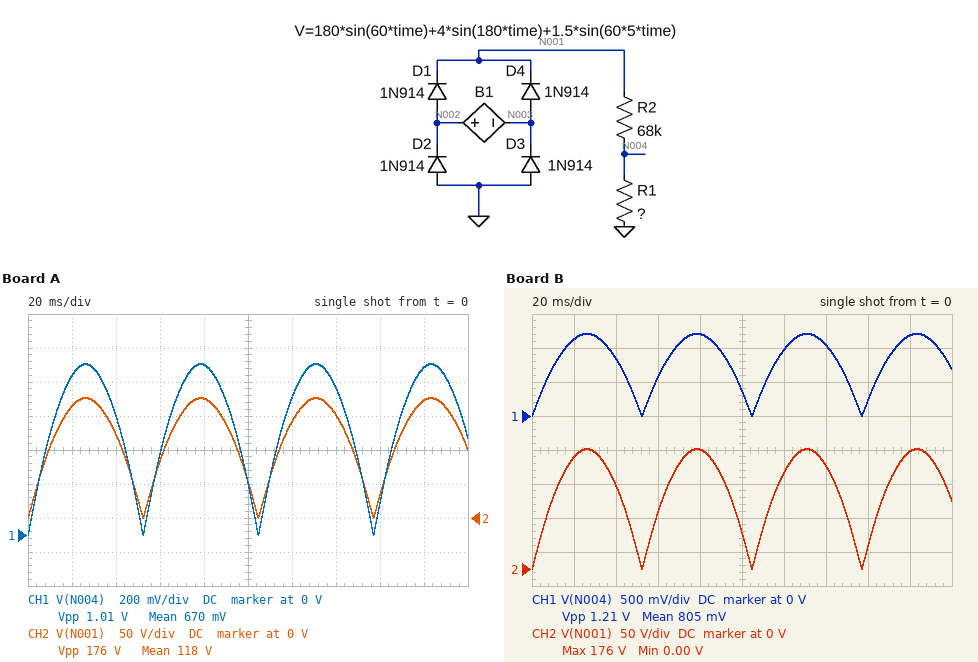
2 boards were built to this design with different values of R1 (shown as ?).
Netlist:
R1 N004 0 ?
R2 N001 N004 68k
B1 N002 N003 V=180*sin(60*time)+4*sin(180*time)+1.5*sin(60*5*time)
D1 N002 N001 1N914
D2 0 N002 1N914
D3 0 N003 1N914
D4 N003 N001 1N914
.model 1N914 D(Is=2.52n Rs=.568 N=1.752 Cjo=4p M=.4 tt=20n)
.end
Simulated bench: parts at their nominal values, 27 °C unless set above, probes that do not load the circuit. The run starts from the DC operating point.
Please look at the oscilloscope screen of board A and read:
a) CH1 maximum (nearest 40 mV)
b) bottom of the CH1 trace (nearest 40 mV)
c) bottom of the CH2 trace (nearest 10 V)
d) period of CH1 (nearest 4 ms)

1.00 V
0 V
0 V
52 ms
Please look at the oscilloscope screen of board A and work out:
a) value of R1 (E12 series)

390 Ω
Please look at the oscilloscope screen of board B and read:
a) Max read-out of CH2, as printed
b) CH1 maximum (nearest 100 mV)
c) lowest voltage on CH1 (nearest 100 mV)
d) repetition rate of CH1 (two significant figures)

176 V
1.2 V
0 V
19 Hz
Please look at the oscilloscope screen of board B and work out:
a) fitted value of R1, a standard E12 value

470 Ω
